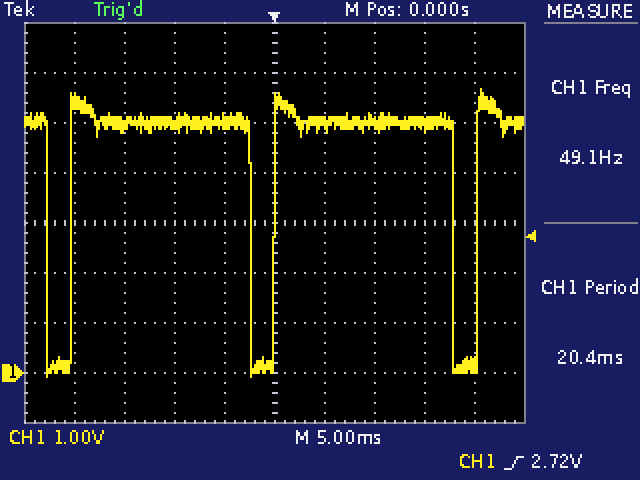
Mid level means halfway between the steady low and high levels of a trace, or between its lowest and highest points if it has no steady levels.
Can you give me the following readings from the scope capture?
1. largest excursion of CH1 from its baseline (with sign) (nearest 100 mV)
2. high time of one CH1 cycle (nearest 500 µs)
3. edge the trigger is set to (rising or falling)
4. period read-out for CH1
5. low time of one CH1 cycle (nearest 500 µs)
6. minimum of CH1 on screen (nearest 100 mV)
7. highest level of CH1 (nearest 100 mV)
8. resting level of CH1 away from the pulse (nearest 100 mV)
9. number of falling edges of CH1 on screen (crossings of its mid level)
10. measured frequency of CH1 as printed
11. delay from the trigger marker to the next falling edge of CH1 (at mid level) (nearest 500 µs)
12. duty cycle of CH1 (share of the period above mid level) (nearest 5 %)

-5.1 V
18.0 ms
rising
20.4 ms
2.5 ms
-100 mV
5.7 V
5.0 V
3
49.1 Hz
18.0 ms
90 %
